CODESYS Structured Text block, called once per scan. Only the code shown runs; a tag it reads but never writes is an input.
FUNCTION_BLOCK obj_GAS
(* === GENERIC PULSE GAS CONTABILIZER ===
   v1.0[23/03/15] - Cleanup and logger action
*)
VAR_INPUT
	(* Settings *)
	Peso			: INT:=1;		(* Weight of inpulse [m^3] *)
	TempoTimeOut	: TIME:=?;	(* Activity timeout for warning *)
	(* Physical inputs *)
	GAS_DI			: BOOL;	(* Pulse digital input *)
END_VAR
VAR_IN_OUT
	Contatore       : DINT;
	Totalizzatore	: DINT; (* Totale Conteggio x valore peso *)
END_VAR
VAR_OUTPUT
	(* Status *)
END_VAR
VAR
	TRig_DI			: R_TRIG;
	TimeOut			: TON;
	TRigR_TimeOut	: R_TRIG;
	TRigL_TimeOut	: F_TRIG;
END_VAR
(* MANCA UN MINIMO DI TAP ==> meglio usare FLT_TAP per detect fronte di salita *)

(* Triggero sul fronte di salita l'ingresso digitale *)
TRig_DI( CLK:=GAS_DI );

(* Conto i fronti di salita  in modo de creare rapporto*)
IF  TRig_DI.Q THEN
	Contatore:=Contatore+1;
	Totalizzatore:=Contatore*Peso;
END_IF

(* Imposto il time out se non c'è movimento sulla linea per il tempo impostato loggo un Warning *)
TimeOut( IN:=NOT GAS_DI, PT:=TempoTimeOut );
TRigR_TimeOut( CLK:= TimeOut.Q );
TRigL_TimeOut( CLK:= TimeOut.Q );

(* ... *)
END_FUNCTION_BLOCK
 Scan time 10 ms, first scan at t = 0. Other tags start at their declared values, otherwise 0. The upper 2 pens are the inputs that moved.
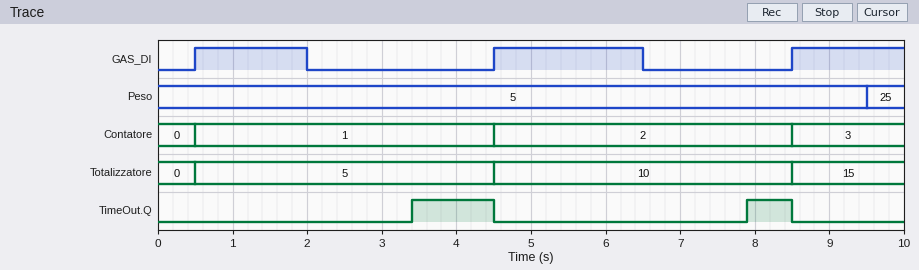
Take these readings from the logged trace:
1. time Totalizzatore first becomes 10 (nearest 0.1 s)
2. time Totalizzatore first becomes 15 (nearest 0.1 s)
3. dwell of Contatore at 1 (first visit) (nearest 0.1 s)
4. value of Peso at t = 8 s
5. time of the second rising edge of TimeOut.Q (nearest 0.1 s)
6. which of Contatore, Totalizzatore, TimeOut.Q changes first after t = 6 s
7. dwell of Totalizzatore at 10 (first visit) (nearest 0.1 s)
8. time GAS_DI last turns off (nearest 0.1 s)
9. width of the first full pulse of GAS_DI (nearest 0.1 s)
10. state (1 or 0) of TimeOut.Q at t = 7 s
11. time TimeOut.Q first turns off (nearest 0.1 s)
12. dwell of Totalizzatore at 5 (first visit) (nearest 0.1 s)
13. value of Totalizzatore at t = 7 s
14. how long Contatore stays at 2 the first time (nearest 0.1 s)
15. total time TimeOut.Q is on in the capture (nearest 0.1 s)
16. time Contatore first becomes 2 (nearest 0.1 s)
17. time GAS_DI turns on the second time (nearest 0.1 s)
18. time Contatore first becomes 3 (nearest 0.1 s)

4.5 s
8.5 s
4.0 s
5
7.9 s
TimeOut.Q
4.0 s
6.5 s
1.5 s
0
4.5 s
4.0 s
10
4.0 s
1.7 s
4.5 s
4.5 s
8.5 s
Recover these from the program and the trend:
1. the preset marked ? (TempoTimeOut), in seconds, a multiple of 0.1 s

1.4 s
